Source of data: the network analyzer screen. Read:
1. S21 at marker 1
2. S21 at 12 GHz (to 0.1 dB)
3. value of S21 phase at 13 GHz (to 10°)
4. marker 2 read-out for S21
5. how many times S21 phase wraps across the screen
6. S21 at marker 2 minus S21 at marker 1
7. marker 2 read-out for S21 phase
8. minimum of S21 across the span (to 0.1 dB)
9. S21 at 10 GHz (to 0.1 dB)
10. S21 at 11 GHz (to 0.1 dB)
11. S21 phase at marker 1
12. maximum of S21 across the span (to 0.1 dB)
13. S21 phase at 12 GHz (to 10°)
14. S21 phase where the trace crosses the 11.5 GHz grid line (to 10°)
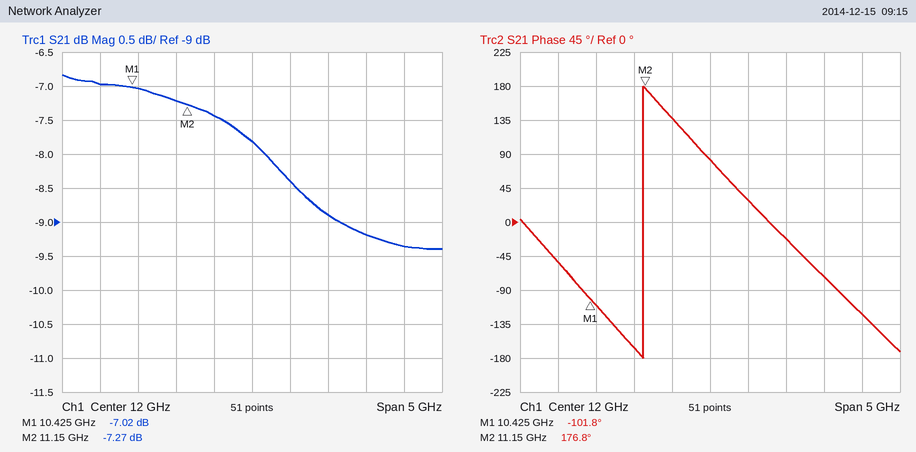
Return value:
-7.02 dB
-7.8 dB
-20°
-7.27 dB
1
-0.25 dB
176.8°
-9.4 dB
-7.0 dB
-7.2 dB
-101.8°
-6.8 dB
80°
140°
